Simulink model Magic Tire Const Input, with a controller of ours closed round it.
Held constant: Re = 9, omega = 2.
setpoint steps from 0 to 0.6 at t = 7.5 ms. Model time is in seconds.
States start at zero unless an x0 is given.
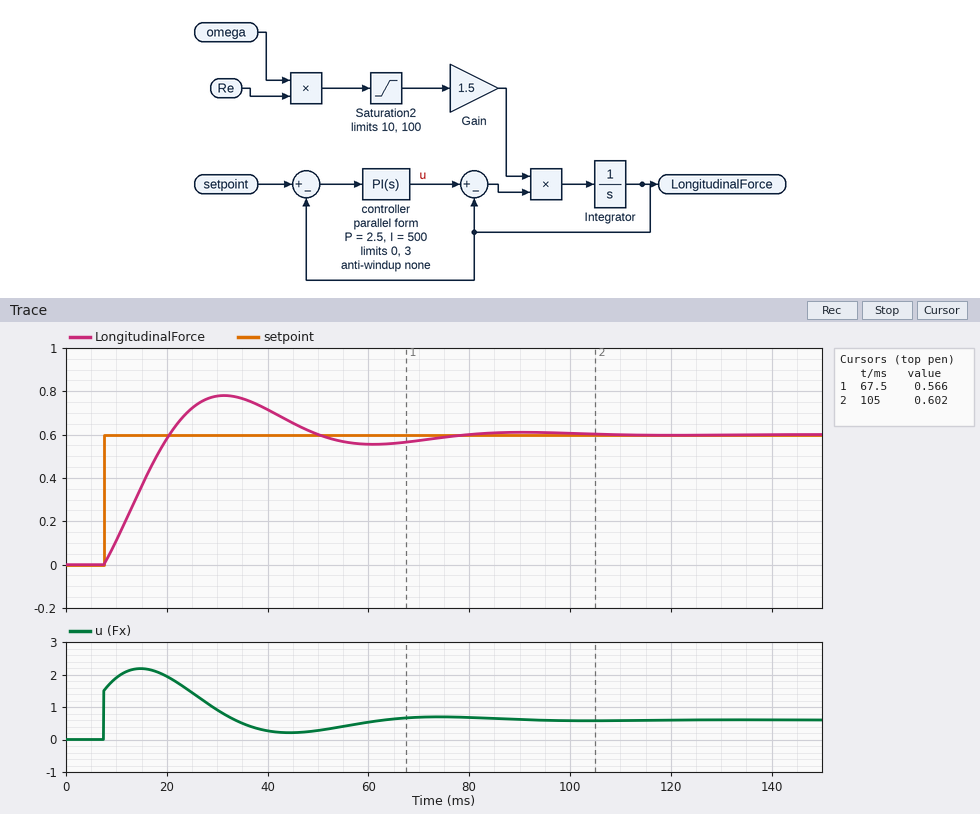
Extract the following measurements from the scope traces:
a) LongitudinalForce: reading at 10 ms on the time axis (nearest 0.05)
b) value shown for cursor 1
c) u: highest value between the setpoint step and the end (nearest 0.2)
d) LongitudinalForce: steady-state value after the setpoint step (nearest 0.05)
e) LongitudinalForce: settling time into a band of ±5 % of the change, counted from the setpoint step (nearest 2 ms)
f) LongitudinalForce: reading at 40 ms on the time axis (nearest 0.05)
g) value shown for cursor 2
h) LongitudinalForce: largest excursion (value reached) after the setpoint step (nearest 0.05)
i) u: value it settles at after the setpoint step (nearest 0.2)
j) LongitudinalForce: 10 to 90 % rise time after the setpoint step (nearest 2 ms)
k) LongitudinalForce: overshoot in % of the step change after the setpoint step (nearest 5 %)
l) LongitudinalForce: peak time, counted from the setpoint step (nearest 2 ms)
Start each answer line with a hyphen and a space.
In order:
- 0.10
- 0.566
- 2.2
- 0.60
- 62 ms
- 0.70
- 0.602
- 0.80
- 0.6
- 10 ms
- 30 %
- 24 ms
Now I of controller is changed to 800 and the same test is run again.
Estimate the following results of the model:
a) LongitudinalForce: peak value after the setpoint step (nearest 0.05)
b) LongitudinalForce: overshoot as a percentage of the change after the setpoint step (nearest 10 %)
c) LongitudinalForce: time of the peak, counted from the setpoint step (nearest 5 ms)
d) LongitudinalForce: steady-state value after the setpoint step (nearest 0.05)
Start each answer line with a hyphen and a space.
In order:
- 0.85
- 40 %
- 20 ms
- 0.60
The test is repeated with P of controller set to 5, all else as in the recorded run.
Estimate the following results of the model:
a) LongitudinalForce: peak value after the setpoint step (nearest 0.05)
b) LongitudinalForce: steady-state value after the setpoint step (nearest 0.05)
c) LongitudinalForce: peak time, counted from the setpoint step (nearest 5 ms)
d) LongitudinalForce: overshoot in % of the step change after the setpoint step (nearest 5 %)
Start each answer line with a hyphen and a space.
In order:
- 0.70
- 0.60
- 20 ms
- 15 %
